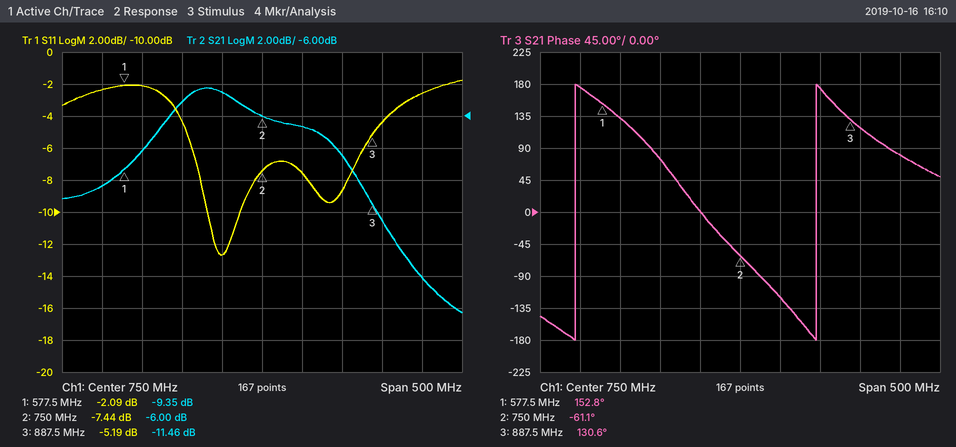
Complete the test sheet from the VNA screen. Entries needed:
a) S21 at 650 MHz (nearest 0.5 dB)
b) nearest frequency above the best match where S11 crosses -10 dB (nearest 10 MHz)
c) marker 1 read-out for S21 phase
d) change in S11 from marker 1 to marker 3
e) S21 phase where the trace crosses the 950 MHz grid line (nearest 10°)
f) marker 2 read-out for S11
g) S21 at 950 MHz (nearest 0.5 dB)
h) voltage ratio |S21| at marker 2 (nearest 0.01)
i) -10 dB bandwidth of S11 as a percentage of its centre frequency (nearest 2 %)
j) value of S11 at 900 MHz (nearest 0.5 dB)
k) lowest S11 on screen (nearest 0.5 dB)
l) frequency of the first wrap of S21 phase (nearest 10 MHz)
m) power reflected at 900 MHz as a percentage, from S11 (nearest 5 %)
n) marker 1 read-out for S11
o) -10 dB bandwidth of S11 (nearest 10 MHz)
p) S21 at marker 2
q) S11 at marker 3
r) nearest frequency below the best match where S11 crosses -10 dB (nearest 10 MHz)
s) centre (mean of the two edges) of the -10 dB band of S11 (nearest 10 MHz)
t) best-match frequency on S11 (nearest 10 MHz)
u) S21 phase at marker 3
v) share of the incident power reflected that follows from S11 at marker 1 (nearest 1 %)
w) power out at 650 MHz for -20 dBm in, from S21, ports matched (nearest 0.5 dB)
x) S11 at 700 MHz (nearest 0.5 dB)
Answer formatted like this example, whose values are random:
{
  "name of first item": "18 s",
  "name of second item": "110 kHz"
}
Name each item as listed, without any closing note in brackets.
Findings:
{
  "S21 at 650 MHz": "-5.0 dB",
  "nearest frequency above the best match where S11 crosses -10 dB": "720 MHz",
  "marker 1 read-out for S21 phase": "152.8°",
  "change in S11 from marker 1 to marker 3": "-3.10 dB",
  "S21 phase where the trace crosses the 950 MHz grid line": "80°",
  "marker 2 read-out for S11": "-7.44 dB",
  "S21 at 950 MHz": "-16.0 dB",
  "voltage ratio |S21| at marker 2": "0.50",
  "-10 dB bandwidth of S11 as a percentage of its centre frequency": "6 %",
  "value of S11 at 900 MHz": "-4.5 dB",
  "lowest S11 on screen": "-12.5 dB",
  "frequency of the first wrap of S21 phase": "540 MHz",
  "power reflected at 900 MHz as a percentage, from S11": "35 %",
  "marker 1 read-out for S11": "-2.09 dB",
  "-10 dB bandwidth of S11": "40 MHz",
  "S21 at marker 2": "-6.00 dB",
  "S11 at marker 3": "-5.19 dB",
  "nearest frequency below the best match where S11 crosses -10 dB": "680 MHz",
  "centre (mean of the two edges) of the -10 dB band of S11": "700 MHz",
  "best-match frequency on S11": "700 MHz",
  "S21 phase at marker 3": "130.6°",
  "share of the incident power reflected that follows from S11 at marker 1": "62 %",
  "power out at 650 MHz for -20 dBm in, from S21, ports matched": "-25.0 dBm",
  "S11 at 700 MHz": "-12.5 dB"
}
